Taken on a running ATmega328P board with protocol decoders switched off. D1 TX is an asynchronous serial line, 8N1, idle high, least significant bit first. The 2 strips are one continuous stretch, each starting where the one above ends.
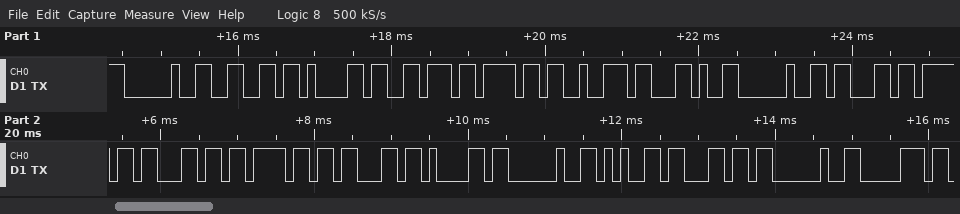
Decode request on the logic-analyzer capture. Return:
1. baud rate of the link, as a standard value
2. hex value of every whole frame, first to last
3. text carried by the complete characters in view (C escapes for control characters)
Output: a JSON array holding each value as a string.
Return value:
["9600 baud", "20 66 61 76 6F 72 2C 20 63 6F 6C 6F 63 61 20 65 6C 20 70", "\" favor, coloca el p\""]
